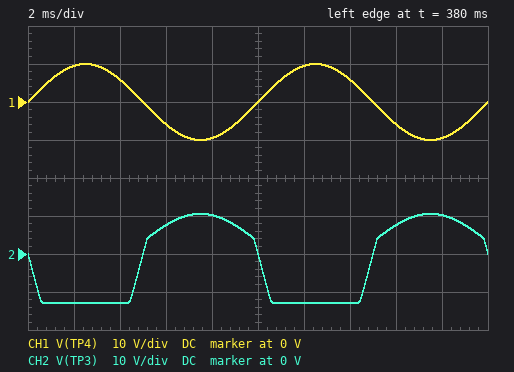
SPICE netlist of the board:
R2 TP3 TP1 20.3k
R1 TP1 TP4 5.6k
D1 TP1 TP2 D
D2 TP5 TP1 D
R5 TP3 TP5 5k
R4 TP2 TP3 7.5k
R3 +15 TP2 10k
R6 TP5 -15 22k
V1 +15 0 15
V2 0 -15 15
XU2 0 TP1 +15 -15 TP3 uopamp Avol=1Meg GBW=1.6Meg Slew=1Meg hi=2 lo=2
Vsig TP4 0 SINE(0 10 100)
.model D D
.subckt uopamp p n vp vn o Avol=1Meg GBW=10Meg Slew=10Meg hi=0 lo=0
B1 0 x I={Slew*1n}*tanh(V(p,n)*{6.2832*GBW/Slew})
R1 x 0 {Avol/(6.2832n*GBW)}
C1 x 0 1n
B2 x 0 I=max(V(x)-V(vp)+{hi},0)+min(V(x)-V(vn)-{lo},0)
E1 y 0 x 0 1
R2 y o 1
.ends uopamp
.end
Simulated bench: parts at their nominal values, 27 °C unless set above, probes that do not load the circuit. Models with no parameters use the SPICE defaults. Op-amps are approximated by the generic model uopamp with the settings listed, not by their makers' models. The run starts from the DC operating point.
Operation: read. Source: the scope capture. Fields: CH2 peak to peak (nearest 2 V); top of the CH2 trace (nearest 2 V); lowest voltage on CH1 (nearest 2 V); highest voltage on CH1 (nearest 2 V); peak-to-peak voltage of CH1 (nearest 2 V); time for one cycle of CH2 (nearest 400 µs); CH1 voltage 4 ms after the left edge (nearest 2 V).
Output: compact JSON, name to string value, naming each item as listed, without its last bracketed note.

{"CH2 peak to peak": "24 V", "top of the CH2 trace": "10 V", "lowest voltage on CH1": "-10 V", "highest voltage on CH1": "10 V", "peak-to-peak voltage of CH1": "20 V", "time for one cycle of CH2": "10.0 ms", "CH1 voltage 4 ms after the left edge": "6 V"}
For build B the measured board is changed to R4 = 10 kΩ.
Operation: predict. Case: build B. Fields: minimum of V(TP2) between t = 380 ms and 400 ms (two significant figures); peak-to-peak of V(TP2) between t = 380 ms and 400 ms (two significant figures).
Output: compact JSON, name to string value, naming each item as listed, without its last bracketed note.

{"minimum of V(TP2) between t = 380 ms and 400 ms": "1.0 V", "peak-to-peak of V(TP2) between t = 380 ms and 400 ms": "12 V"}
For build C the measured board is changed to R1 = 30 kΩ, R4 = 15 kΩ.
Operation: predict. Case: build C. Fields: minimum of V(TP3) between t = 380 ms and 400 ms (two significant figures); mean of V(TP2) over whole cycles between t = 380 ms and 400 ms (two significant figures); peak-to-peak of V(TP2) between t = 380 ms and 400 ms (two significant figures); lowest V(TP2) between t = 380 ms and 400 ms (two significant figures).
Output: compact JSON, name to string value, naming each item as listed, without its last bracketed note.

{"minimum of V(TP3) between t = 380 ms and 400 ms": "-6.8 V", "mean of V(TP2) over whole cycles between t = 380 ms and 400 ms": "8.8 V", "peak-to-peak of V(TP2) between t = 380 ms and 400 ms": "4.6 V", "lowest V(TP2) between t = 380 ms and 400 ms": "6.3 V"}
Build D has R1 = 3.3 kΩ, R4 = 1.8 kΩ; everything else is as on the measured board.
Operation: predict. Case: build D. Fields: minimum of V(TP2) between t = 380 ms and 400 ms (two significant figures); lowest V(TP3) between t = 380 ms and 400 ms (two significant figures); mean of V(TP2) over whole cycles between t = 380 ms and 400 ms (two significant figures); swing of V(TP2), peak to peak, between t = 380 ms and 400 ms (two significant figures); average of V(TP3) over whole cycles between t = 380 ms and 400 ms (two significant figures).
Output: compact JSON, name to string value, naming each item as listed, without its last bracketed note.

{"minimum of V(TP2) between t = 380 ms and 400 ms": "-680 mV", "lowest V(TP3) between t = 380 ms and 400 ms": "-8.2 V", "mean of V(TP2) over whole cycles between t = 380 ms and 400 ms": "5.2 V", "swing of V(TP2), peak to peak, between t = 380 ms and 400 ms": "14 V", "average of V(TP3) over whole cycles between t = 380 ms and 400 ms": "2.0 V"}
